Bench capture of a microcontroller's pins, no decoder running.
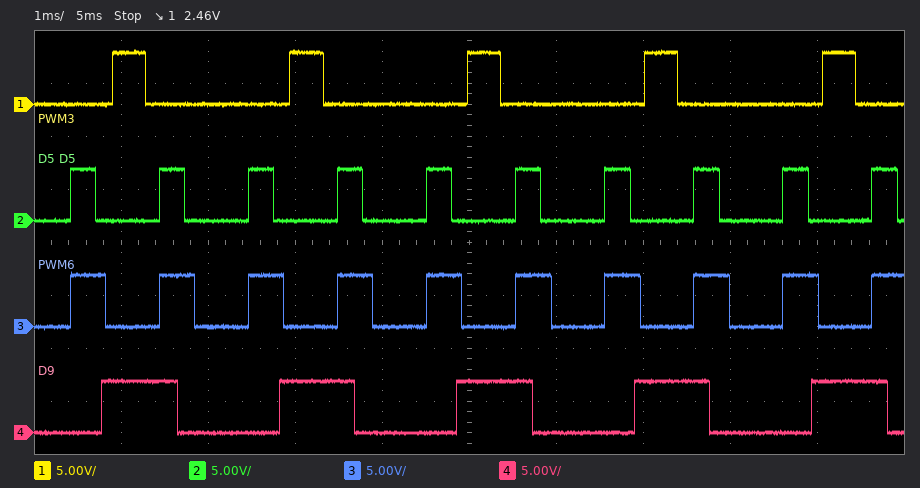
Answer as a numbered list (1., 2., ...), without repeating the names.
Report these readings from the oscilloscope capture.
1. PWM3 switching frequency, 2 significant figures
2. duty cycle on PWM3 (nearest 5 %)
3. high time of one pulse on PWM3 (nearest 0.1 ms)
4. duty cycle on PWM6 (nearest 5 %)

1. 490 Hz
2. 20 %
3. 0.4 ms
4. 40 %
